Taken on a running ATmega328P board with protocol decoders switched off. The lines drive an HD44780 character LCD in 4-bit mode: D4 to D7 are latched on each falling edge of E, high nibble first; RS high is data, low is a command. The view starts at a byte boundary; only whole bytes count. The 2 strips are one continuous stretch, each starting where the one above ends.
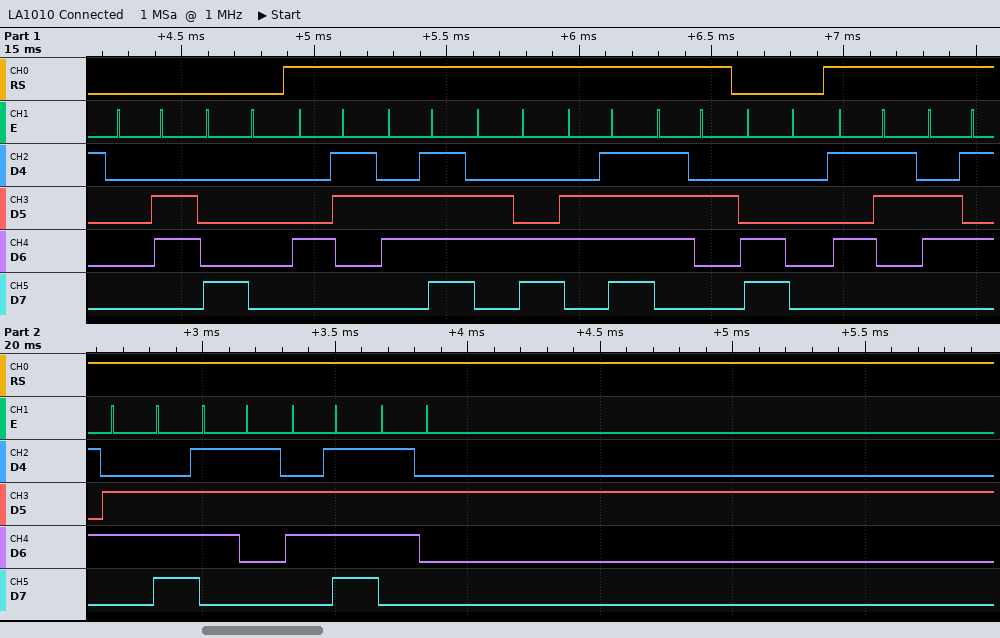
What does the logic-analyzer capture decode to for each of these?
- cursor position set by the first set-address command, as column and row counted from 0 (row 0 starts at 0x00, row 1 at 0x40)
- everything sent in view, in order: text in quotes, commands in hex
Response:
column 0, row 0
0x06 0x80 "Color" 0xC0 "Sensor"
